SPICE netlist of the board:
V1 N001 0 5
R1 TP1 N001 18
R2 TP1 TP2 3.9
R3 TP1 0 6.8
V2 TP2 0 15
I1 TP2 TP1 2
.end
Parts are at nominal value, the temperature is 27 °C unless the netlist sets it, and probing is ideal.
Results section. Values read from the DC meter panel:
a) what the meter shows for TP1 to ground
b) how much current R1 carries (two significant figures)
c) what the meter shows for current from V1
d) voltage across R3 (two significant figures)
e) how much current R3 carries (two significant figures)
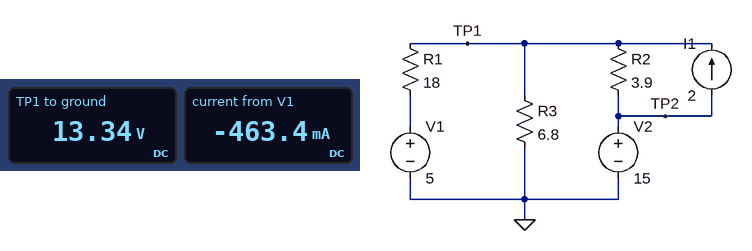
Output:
13.34 V
460 mA
-463.4 mA
13 V
2.0 A
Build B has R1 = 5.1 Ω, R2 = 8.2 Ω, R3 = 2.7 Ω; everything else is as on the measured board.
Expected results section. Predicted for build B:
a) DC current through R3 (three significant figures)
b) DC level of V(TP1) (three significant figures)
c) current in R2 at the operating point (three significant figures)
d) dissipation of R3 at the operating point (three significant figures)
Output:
2.59 A
6.99 V
977 mA
18.1 W
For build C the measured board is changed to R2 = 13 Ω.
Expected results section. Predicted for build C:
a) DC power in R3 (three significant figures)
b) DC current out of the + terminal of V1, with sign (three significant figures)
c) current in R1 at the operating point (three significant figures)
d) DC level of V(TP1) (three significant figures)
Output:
22.2 W
-404 mA
404 mA
12.3 V
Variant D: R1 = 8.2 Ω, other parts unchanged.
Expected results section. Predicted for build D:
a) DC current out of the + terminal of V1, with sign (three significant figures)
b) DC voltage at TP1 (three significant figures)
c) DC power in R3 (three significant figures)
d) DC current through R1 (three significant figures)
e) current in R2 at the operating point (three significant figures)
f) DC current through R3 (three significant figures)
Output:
-889 mA
12.3 V
22.2 W
889 mA
696 mA
1.81 A
